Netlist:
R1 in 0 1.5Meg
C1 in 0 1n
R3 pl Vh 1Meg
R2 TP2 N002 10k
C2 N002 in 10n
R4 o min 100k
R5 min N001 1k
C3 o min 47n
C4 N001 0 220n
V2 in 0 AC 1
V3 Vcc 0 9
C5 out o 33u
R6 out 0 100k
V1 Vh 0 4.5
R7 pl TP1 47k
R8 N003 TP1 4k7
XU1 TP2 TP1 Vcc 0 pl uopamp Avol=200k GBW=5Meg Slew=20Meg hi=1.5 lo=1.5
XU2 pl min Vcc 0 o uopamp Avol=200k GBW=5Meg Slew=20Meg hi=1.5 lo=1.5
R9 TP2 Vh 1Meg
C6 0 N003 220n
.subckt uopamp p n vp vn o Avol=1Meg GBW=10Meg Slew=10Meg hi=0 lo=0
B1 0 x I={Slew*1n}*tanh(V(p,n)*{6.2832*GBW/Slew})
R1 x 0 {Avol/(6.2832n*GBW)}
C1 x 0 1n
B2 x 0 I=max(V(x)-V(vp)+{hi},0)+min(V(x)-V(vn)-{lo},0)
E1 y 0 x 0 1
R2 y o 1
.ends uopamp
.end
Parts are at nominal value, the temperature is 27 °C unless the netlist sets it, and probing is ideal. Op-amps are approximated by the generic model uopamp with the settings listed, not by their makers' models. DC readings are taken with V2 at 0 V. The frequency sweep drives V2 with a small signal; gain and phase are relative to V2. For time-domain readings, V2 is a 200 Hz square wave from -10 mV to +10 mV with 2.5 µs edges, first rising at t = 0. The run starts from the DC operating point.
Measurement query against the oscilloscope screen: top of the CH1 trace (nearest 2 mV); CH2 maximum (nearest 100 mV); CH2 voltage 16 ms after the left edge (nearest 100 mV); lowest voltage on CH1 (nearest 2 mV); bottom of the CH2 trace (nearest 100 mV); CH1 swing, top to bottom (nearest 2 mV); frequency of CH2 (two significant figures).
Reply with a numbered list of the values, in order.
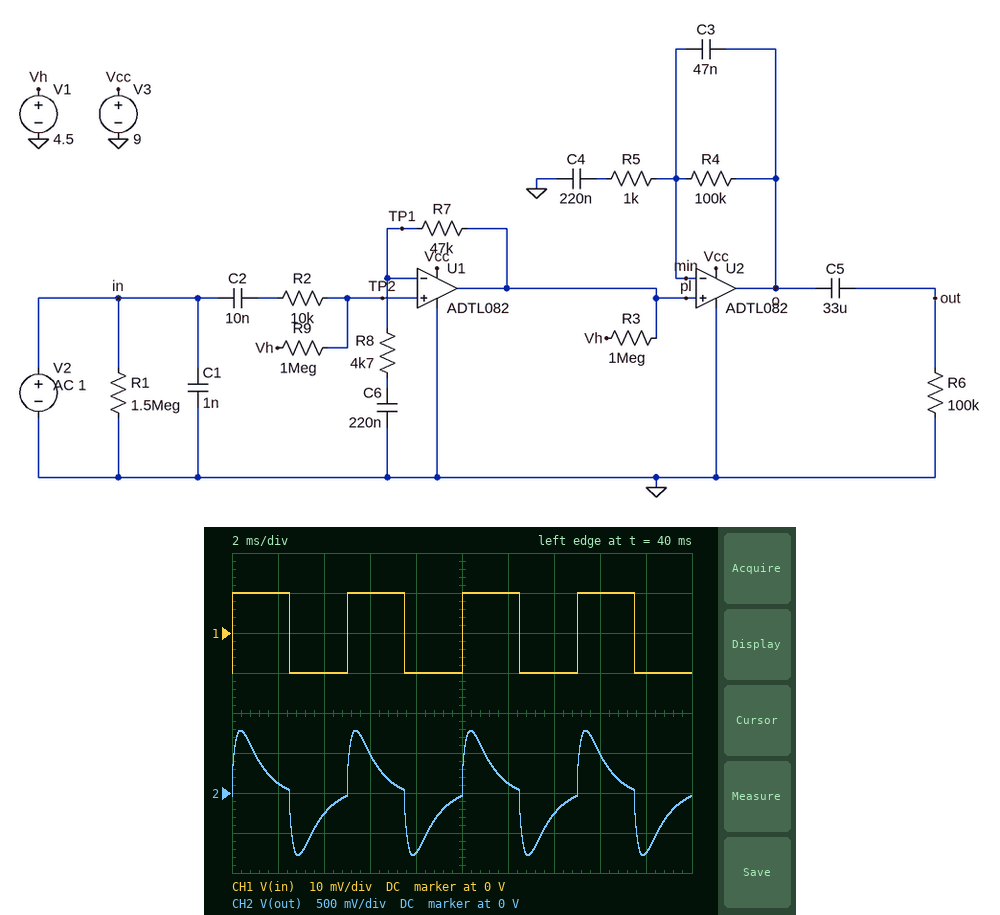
1. 10 mV
2. 800 mV
3. 500 mV
4. -10 mV
5. -800 mV
6. 20 mV
7. 200 Hz
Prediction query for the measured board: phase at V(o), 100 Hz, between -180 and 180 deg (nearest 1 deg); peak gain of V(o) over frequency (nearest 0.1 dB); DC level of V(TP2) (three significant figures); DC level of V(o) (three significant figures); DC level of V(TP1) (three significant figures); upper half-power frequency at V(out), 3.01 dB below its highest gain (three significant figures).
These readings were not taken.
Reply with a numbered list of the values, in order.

1. 67 deg
2. 34.2 dB
3. 4.50 V
4. 4.50 V
5. 4.50 V
6. 1.04 kHz
